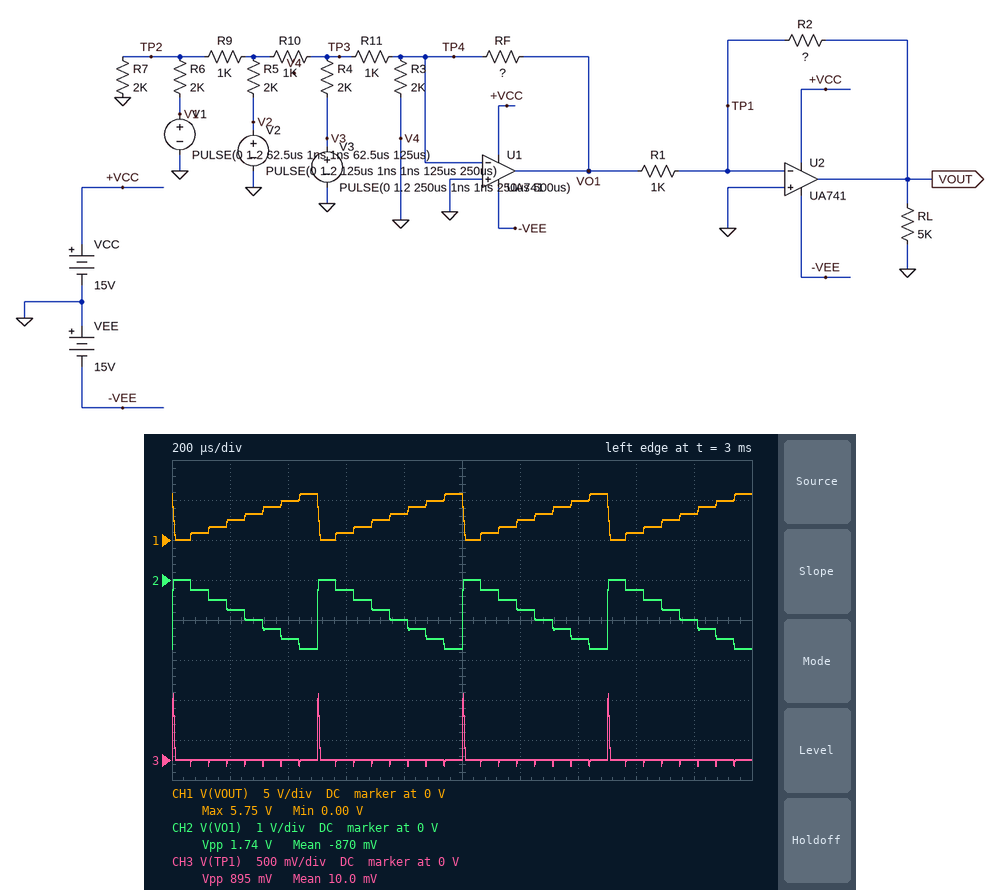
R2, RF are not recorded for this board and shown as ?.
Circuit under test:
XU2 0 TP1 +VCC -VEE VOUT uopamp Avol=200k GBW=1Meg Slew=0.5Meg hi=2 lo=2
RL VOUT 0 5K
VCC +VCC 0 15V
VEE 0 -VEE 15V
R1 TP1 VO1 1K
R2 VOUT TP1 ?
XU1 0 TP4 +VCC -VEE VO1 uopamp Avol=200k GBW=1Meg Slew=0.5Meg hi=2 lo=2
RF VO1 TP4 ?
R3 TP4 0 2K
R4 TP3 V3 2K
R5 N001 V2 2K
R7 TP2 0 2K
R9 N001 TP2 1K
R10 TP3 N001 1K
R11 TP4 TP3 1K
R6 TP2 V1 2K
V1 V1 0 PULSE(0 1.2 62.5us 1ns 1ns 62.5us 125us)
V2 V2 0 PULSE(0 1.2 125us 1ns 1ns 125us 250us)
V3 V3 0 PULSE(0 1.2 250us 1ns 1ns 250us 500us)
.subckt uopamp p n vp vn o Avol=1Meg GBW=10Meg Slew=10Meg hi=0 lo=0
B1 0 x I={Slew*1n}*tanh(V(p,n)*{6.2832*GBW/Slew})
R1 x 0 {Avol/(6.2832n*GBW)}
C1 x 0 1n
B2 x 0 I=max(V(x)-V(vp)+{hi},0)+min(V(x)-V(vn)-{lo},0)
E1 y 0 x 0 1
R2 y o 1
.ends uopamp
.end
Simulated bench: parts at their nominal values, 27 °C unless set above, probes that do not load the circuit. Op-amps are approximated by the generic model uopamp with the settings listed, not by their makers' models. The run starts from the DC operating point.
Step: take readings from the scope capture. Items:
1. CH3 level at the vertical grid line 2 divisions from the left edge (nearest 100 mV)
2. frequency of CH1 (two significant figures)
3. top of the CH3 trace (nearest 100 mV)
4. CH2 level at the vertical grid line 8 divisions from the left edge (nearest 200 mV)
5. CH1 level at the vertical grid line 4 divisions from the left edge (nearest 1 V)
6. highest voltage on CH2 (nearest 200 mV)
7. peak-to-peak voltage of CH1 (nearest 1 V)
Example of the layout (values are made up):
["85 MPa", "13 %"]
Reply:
["0 V", "2.0 kHz", "800 mV", "-200 mV", "3 V", "0 V", "6 V"]
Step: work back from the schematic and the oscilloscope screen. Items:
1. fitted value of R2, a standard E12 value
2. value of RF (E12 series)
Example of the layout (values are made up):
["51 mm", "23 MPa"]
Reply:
["3.3 kΩ", "3.3 kΩ"]
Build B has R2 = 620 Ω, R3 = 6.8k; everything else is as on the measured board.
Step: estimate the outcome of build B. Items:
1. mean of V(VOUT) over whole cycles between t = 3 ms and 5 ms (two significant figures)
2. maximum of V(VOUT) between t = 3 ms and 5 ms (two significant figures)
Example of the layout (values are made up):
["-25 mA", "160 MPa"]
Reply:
["540 mV", "1.1 V"]
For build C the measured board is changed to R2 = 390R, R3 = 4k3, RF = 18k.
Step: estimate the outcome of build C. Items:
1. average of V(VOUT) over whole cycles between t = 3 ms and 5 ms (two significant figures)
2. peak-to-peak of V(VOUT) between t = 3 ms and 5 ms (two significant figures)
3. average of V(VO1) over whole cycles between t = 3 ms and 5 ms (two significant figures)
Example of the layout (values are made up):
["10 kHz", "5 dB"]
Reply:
["1.9 V", "3.7 V", "-4.9 V"]
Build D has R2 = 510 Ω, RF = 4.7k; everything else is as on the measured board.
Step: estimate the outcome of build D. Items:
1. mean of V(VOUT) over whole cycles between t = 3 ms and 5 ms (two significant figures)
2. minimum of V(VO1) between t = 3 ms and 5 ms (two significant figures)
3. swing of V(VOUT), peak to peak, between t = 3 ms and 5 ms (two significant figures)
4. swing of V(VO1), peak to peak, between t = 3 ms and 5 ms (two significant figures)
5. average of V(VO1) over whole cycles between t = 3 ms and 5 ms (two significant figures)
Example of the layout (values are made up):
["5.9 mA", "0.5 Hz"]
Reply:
["630 mV", "-2.5 V", "1.3 V", "2.5 V", "-1.2 V"]
